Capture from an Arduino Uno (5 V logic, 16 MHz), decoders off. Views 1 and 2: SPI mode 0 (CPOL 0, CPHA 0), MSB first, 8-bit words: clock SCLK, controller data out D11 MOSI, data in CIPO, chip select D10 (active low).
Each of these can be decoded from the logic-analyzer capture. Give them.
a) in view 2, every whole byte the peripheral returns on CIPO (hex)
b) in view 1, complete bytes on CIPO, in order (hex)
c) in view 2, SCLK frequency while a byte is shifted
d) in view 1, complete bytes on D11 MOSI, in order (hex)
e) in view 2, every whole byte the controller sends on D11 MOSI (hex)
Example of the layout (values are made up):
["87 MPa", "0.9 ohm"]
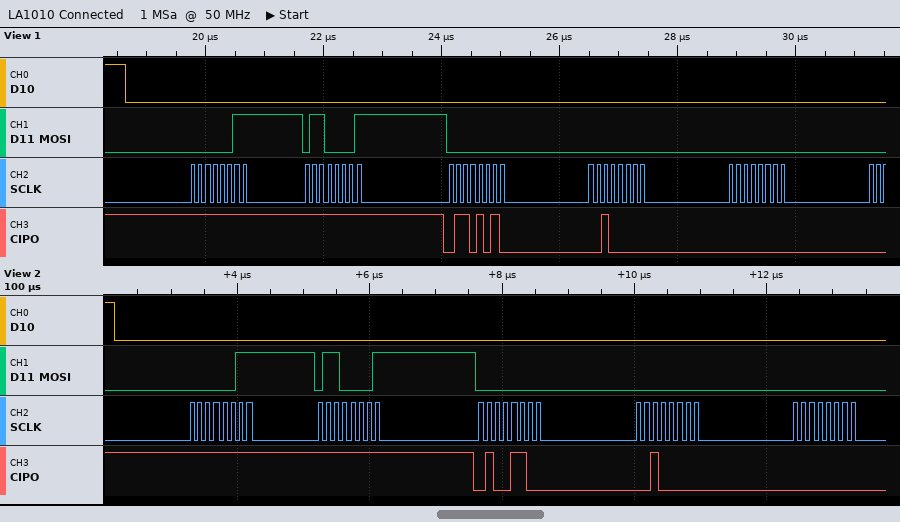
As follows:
["FF FF 4C 20 00", "FF FF 6A 20 00", "8 MHz", "03 61 00 00 00", "03 61 00 00 00"]
